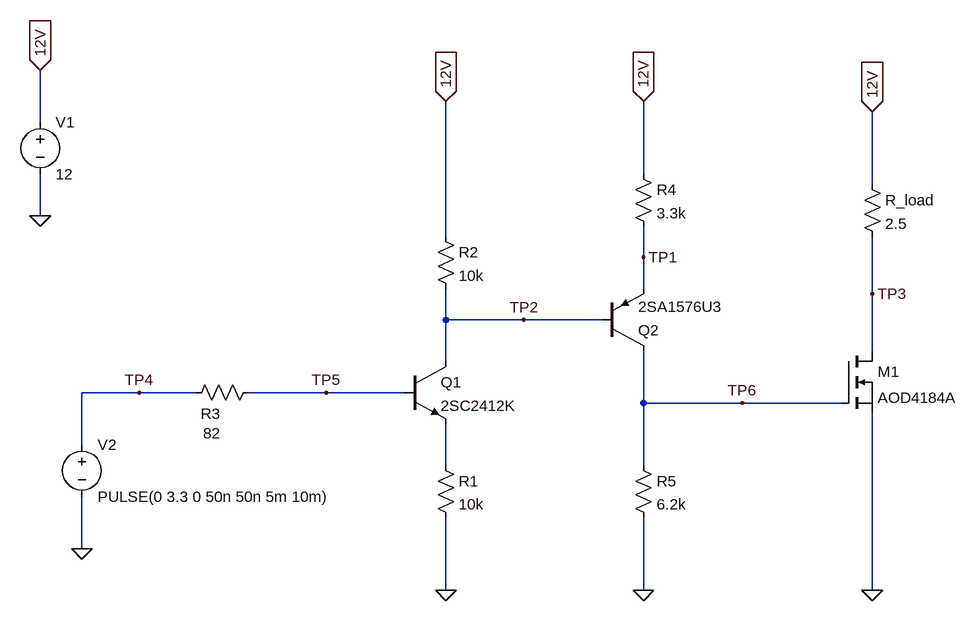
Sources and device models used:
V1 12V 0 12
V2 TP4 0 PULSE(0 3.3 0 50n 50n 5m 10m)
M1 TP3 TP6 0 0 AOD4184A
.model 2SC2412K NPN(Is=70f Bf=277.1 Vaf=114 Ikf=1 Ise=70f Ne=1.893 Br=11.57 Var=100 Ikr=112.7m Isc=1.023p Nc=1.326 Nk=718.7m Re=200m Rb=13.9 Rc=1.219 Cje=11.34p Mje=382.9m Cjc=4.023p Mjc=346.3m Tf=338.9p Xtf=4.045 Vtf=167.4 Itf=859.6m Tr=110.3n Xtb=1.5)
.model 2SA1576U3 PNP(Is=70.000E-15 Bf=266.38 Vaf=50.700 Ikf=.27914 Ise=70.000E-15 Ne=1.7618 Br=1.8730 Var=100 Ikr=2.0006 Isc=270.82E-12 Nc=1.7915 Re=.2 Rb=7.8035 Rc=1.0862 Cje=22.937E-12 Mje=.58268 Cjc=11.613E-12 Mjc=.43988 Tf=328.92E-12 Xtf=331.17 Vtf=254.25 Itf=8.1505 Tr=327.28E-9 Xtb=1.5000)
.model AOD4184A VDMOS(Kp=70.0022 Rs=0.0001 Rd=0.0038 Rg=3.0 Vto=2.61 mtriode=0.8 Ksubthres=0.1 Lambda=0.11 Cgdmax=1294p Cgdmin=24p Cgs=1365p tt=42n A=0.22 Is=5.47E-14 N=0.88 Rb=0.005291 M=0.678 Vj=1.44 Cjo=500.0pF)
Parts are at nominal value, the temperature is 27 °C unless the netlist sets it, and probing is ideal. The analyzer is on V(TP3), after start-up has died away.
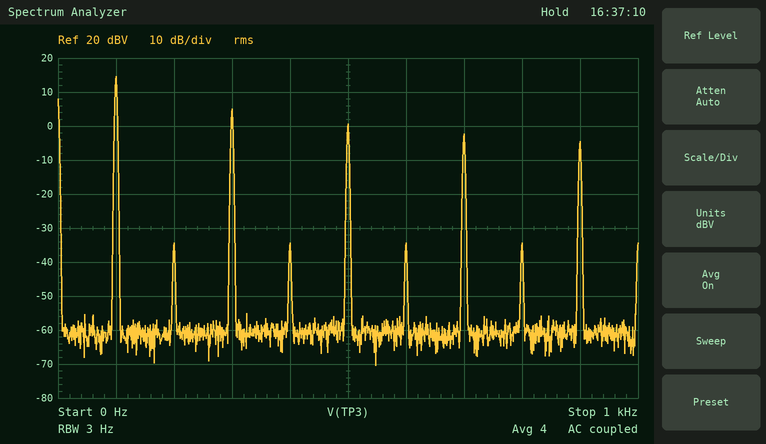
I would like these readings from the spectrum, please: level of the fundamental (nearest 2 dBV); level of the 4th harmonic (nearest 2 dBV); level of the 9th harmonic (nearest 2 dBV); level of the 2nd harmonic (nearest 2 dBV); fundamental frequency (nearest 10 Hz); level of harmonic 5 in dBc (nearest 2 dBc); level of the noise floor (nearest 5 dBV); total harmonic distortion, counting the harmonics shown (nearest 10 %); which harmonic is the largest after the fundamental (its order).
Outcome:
14 dBV
-34 dBV
-4 dBV
-34 dBV
100 Hz
-14 dBc
-60 dBV
40 %
3
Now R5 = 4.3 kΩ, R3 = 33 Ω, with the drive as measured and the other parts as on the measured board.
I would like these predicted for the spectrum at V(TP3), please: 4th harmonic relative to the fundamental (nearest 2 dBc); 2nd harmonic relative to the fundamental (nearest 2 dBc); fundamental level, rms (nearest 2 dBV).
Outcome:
-34 dBc
-34 dBc
4 dBV
